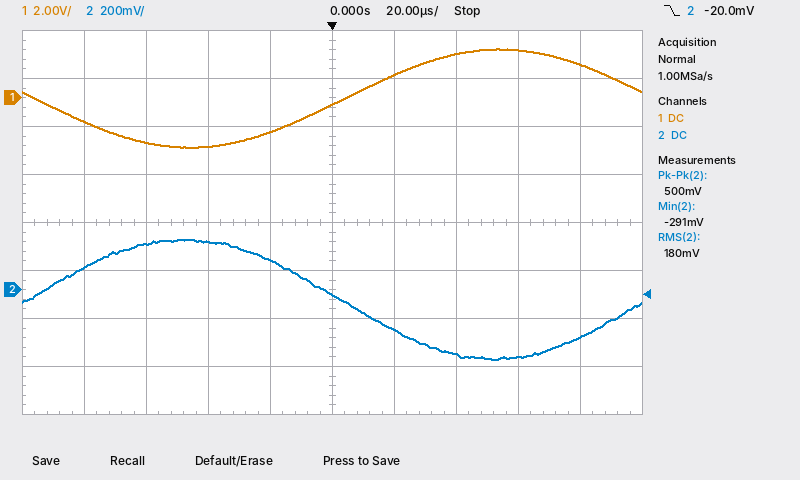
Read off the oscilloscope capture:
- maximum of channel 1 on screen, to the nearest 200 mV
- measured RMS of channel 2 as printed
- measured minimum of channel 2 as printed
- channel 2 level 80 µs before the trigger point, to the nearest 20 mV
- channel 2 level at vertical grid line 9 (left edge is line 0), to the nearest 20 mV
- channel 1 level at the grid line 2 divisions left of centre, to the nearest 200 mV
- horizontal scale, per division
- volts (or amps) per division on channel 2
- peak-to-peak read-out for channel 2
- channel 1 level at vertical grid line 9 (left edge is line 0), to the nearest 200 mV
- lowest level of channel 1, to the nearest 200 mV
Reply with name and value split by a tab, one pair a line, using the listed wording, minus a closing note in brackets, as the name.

maximum of channel 1 on screen, to the nearest 200 mV	2.0 V
measured RMS of channel 2 as printed	180 mV
measured minimum of channel 2 as printed	-291 mV
channel 2 level 80 µs before the trigger point, to the nearest 20 mV	100 mV
channel 2 level at vertical grid line 9 (left edge is line 0), to the nearest 20 mV	-200 mV
channel 1 level at the grid line 2 divisions left of centre, to the nearest 200 mV	-2.0 V
horizontal scale, per division	20 µs
volts (or amps) per division on channel 2	200 mV
peak-to-peak read-out for channel 2	500 mV
channel 1 level at vertical grid line 9 (left edge is line 0), to the nearest 200 mV	1.4 V
lowest level of channel 1, to the nearest 200 mV	-2.0 V
